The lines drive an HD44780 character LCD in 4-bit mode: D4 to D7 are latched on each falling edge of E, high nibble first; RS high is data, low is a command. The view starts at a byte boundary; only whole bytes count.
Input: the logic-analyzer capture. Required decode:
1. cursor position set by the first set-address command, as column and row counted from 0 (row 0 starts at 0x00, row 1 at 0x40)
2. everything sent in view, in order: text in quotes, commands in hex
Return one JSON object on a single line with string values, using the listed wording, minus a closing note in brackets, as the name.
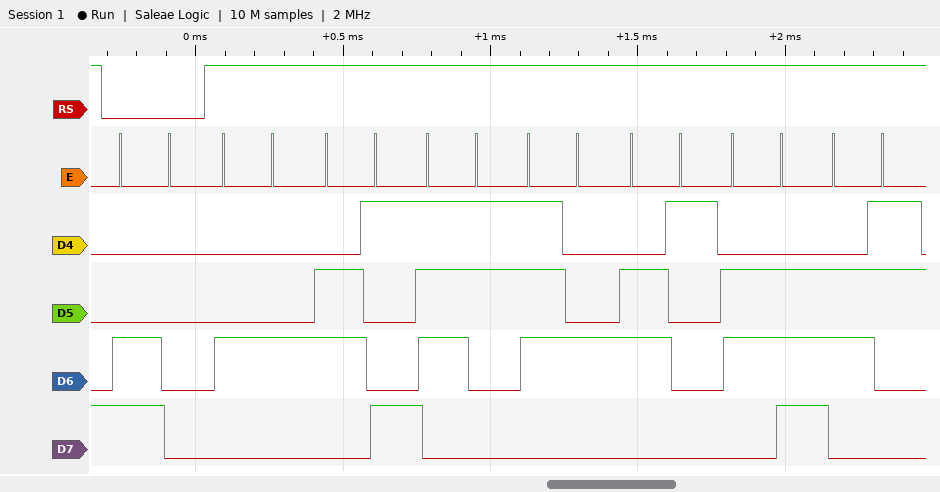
{"cursor position set by the first set-address command, as column and row counted from 0": "column 0, row 1", "everything sent in view, in order: text in quotes, commands in hex": "0xC0 \"Distanc\""}
